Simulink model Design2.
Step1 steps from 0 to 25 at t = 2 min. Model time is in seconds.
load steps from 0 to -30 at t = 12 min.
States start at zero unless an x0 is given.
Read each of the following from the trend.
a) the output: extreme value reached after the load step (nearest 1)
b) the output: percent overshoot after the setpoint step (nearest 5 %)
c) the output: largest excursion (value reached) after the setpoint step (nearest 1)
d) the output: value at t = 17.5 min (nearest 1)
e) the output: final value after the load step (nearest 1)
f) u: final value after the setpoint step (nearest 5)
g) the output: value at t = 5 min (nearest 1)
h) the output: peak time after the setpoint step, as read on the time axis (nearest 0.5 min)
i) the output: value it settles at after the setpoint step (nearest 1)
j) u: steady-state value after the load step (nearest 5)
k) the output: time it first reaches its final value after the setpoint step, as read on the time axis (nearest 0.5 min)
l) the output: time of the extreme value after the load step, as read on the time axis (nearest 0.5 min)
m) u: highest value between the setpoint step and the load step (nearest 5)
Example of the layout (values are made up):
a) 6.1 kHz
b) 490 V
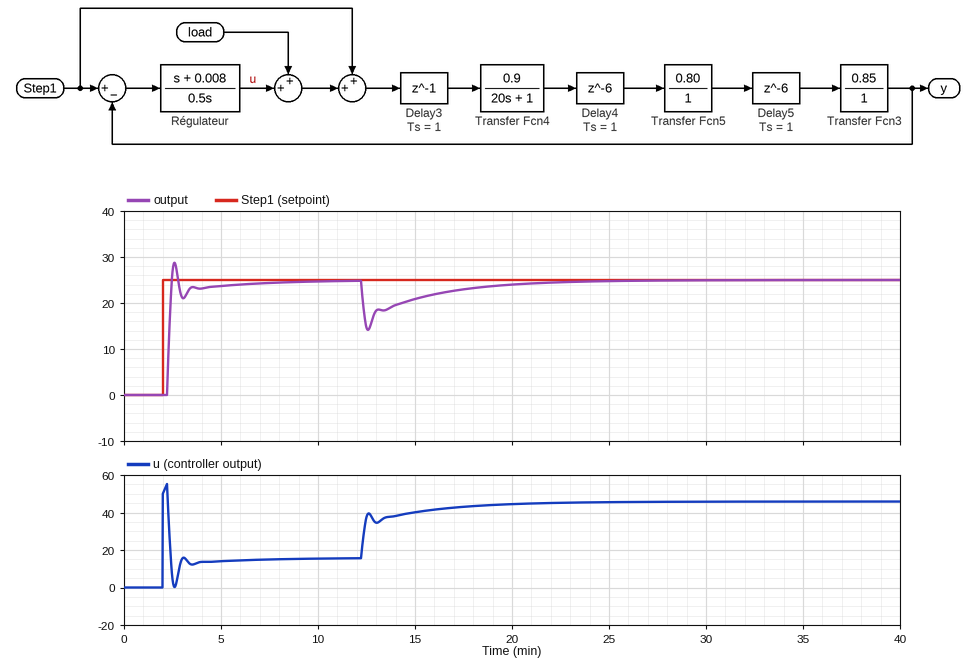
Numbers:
a) 14
b) 15 %
c) 29
d) 23
e) 25
f) 15
g) 24
h) 2.5 min
i) 25
j) 45
k) 2.5 min
l) 12.5 min
m) 55
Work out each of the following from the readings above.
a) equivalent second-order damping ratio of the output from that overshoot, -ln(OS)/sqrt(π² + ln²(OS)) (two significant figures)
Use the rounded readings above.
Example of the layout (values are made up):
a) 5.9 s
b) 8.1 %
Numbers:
a) 0.52
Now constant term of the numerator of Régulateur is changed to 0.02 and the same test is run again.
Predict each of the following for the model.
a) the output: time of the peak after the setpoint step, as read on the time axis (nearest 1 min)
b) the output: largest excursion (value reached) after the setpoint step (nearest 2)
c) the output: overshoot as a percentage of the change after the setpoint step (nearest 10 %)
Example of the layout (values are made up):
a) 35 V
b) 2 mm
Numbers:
a) 3 min
b) 32
c) 30 %
